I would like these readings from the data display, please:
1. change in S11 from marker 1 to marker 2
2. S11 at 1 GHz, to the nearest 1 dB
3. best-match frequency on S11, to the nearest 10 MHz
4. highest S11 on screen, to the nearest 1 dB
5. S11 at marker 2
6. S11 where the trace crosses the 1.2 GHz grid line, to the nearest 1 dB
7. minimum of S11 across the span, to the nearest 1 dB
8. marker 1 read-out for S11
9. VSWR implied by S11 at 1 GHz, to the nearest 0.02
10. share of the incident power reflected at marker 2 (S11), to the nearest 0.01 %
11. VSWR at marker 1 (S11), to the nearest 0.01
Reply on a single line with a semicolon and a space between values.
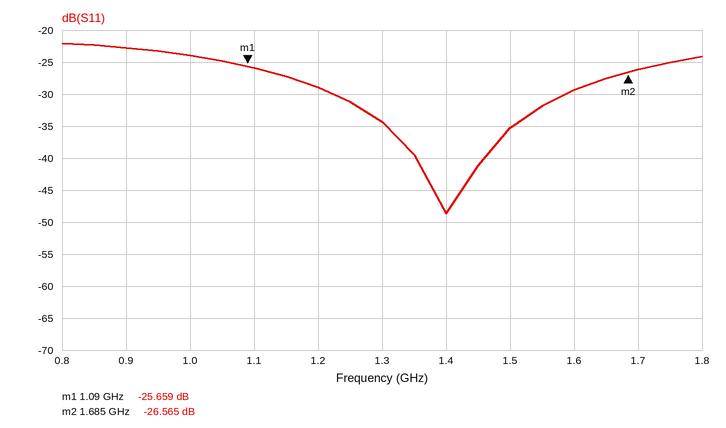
-0.906 dB; -24 dB; 1.40 GHz; -22 dB; -26.565 dB; -29 dB; -49 dB; -25.659 dB; 1.14; 0.22 %; 1.11
